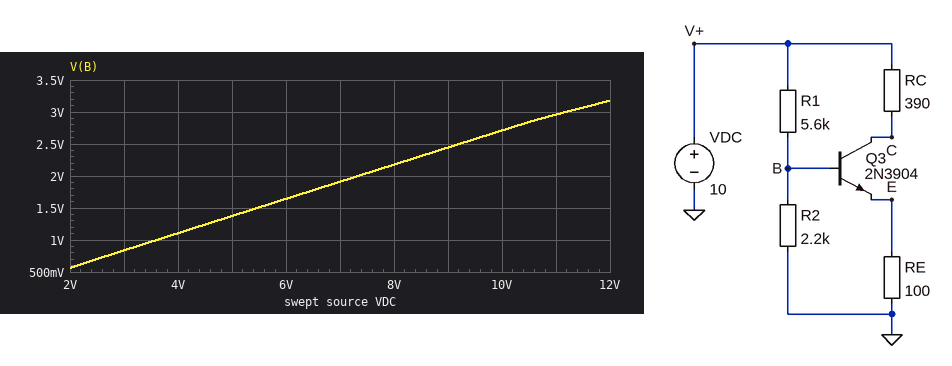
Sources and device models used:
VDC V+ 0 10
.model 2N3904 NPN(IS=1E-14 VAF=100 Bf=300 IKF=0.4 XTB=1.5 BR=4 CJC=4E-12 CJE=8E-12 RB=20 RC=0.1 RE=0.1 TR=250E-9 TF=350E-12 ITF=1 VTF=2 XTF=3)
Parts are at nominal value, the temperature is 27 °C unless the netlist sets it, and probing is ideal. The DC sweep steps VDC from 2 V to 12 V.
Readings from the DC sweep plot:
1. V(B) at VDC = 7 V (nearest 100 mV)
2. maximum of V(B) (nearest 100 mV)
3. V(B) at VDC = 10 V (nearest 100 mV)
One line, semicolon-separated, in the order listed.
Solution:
1.9 V; 3.2 V; 2.7 V
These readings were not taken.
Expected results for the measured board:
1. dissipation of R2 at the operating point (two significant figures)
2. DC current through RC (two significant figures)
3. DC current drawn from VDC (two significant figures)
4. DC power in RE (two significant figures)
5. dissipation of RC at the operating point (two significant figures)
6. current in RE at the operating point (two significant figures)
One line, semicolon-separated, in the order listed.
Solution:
3.3 mW; 20 mA; 21 mA; 39 mW; 150 mW; 20 mA
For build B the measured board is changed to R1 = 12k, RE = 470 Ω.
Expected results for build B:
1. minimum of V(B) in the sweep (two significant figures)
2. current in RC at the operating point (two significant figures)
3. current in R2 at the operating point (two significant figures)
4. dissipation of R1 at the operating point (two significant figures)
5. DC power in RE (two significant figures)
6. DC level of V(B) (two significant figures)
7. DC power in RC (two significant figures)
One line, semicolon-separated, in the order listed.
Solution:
310 mV; 1.8 mA; 700 µA; 6.0 mW; 1.6 mW; 1.5 V; 1.3 mW
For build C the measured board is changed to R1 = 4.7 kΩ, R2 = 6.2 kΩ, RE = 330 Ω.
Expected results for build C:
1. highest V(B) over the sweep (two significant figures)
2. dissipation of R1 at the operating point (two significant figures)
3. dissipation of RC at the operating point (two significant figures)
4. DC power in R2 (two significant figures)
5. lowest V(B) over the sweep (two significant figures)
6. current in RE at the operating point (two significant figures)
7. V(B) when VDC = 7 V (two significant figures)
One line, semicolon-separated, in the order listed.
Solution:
6.2 V; 4.7 mW; 73 mW; 4.5 mW; 1.1 V; 14 mA; 3.9 V
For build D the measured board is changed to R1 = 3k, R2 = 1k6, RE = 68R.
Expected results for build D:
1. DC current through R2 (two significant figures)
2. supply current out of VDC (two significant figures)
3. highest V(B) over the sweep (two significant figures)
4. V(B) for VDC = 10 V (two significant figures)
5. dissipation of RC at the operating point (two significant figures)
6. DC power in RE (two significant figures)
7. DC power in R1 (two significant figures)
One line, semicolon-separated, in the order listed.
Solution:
1.4 mA; 24 mA; 2.6 V; 2.3 V; 180 mW; 35 mW; 20 mW
